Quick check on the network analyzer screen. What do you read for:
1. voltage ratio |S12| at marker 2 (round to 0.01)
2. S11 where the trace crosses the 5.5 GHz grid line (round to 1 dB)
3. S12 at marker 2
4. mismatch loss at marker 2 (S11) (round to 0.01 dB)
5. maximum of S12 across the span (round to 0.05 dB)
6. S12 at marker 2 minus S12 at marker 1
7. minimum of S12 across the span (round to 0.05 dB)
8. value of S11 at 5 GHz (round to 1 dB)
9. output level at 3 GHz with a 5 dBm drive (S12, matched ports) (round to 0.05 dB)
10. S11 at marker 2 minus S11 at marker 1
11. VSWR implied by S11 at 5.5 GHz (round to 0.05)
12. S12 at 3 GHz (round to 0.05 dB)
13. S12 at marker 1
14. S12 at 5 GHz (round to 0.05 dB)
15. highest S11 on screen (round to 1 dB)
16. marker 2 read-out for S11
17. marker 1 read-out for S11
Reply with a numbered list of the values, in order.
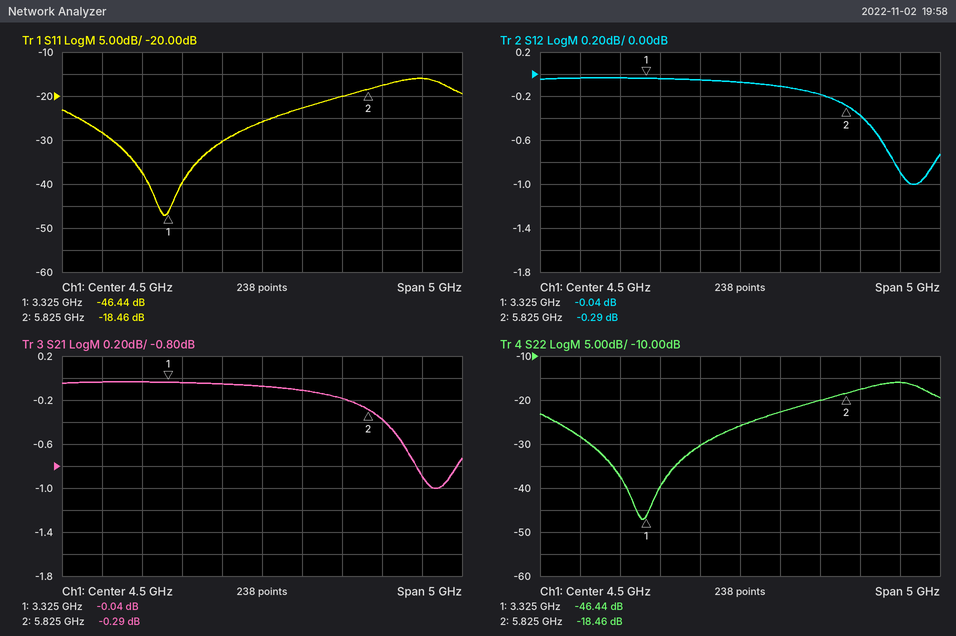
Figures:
1. 0.97
2. -20 dB
3. -0.29 dB
4. 0.06 dB
5. -0.05 dB
6. -0.25 dB
7. -1.00 dB
8. -23 dB
9. 4.95 dBm
10. 27.98 dB
11. 1.20
12. -0.05 dB
13. -0.04 dB
14. -0.10 dB
15. -16 dB
16. -18.46 dB
17. -46.44 dB
